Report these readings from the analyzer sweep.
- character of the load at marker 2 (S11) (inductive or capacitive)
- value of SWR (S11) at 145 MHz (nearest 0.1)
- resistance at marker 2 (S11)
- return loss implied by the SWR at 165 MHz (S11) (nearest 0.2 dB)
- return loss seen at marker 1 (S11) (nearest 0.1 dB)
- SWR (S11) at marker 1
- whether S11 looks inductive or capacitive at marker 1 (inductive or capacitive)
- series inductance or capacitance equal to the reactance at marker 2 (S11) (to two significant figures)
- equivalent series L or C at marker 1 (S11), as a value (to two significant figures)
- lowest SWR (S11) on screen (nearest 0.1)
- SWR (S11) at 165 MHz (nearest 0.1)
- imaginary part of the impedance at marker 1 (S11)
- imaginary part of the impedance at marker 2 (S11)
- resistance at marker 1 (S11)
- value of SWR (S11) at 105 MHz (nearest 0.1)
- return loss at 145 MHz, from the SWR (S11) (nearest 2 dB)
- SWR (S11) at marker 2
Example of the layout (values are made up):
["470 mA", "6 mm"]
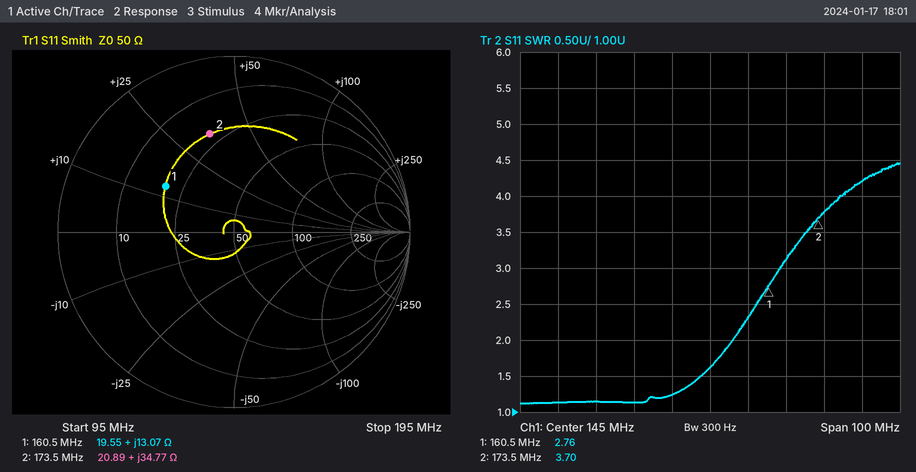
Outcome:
["inductive", "1.6", "20.89 Ω", "5.8 dB", "6.6 dB", "2.76", "inductive", "32 nH", "13 nH", "1.1", "3.1", "+13.07 Ω", "+34.77 Ω", "19.55 Ω", "1.1", "12 dB", "3.70"]
